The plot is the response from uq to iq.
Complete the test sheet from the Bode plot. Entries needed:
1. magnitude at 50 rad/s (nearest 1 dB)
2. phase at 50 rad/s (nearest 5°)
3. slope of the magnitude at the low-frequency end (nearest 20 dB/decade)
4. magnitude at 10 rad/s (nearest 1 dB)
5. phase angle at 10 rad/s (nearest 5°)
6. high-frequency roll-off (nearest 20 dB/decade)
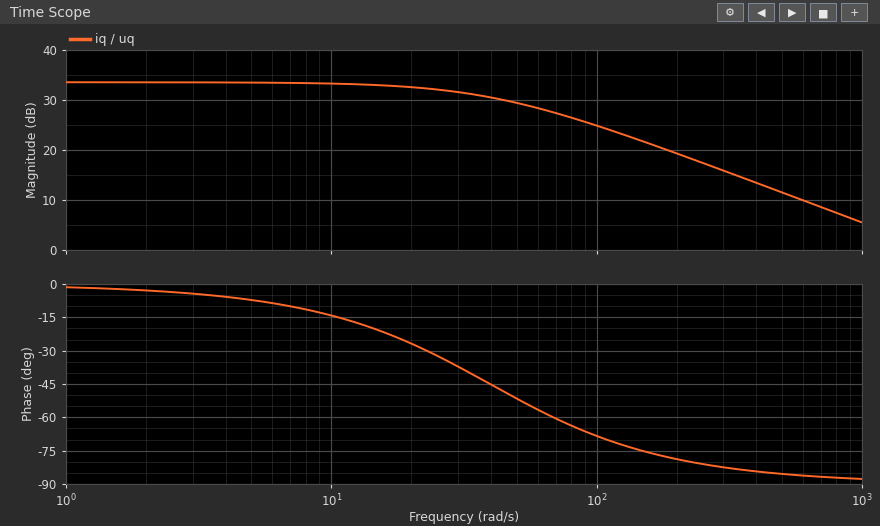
29 dB
-50°
0 dB/decade
33 dB
-15°
-20 dB/decade
